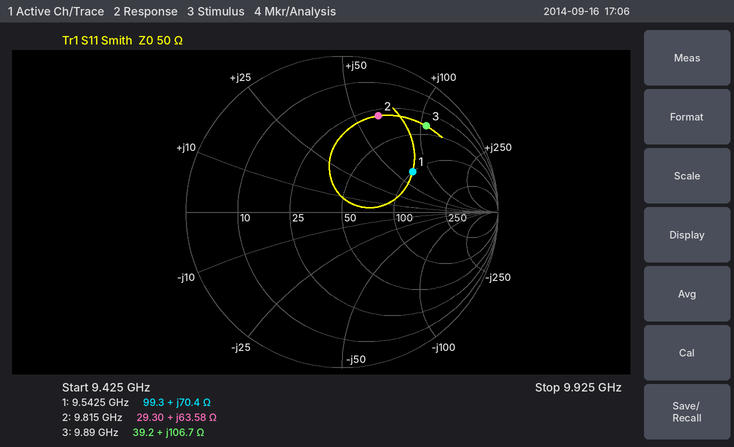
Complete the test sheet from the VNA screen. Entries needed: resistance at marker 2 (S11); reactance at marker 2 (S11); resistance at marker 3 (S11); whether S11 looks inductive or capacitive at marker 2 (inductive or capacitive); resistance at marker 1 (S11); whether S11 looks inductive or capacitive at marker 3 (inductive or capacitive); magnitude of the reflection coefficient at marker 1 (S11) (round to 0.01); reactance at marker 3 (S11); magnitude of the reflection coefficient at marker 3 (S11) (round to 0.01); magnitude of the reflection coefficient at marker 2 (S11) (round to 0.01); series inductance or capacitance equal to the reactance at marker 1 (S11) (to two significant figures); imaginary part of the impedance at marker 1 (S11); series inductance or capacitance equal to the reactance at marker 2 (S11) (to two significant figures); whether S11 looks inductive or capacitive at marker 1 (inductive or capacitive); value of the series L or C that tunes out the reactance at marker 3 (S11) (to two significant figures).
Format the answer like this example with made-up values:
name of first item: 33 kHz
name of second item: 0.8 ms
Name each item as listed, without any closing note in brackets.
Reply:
resistance at marker 2: 29.30 Ω
reactance at marker 2: +63.58 Ω
resistance at marker 3: 39.2 Ω
whether S11 looks inductive or capacitive at marker 2: inductive
resistance at marker 1: 99.3 Ω
whether S11 looks inductive or capacitive at marker 3: inductive
magnitude of the reflection coefficient at marker 1 (S11): 0.52
reactance at marker 3: +106.7 Ω
magnitude of the reflection coefficient at marker 3 (S11): 0.77
magnitude of the reflection coefficient at marker 2 (S11): 0.66
series inductance or capacitance equal to the reactance at marker 1 (S11): 1.2 nH
imaginary part of the impedance at marker 1: +70.4 Ω
series inductance or capacitance equal to the reactance at marker 2 (S11): 1.0 nH
whether S11 looks inductive or capacitive at marker 1: inductive
value of the series L or C that tunes out the reactance at marker 3 (S11): 150 fF
